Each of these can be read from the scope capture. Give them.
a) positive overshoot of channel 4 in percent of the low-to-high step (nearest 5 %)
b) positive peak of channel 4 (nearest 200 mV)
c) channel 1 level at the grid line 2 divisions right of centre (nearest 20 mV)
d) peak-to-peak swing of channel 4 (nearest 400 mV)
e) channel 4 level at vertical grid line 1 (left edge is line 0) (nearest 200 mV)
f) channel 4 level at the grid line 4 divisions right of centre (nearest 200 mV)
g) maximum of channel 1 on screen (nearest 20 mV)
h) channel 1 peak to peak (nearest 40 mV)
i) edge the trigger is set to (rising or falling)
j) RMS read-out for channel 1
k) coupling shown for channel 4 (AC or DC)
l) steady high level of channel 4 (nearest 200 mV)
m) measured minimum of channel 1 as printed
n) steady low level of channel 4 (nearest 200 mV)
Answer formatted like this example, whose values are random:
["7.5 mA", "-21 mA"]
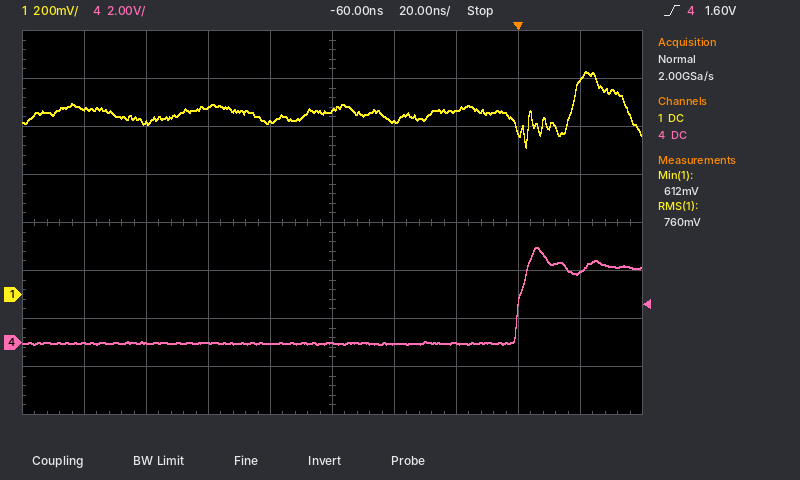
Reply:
["25 %", "4.0 V", "760 mV", "4.0 V", "0.0 V", "3.0 V", "920 mV", "320 mV", "rising", "760 mV", "DC", "3.2 V", "612 mV", "0.0 V"]
